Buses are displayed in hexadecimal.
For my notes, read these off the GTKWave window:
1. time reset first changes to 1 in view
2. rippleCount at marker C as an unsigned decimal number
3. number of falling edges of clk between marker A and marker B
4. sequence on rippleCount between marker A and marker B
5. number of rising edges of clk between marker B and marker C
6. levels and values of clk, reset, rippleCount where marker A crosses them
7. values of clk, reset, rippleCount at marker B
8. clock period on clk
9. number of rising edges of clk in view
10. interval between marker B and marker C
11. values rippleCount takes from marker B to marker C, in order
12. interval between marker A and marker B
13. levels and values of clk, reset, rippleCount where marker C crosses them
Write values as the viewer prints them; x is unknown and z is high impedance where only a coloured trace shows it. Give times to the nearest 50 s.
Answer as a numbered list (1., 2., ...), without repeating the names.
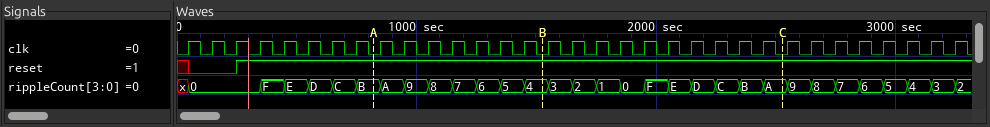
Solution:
1. 250 s
2. 10
3. 7
4. B, A, 9, 8, 7, 6, 5, 4
5. 10
6. clk=0, reset=1, rippleCount=B
7. clk=0, reset=1, rippleCount=4
8. 100 s
9. 33
10. 1000 s
11. 4, 3, 2, 1, 0, F, E, D, C, B, A
12. 700 s
13. clk=0, reset=1, rippleCount=A
